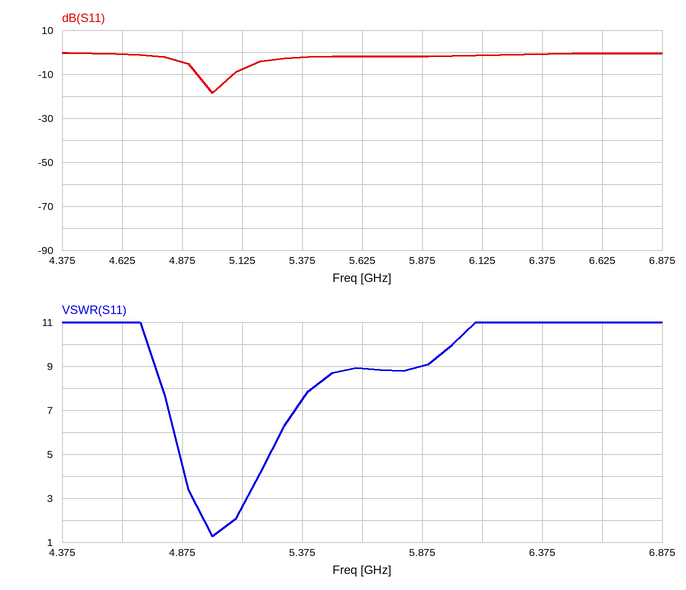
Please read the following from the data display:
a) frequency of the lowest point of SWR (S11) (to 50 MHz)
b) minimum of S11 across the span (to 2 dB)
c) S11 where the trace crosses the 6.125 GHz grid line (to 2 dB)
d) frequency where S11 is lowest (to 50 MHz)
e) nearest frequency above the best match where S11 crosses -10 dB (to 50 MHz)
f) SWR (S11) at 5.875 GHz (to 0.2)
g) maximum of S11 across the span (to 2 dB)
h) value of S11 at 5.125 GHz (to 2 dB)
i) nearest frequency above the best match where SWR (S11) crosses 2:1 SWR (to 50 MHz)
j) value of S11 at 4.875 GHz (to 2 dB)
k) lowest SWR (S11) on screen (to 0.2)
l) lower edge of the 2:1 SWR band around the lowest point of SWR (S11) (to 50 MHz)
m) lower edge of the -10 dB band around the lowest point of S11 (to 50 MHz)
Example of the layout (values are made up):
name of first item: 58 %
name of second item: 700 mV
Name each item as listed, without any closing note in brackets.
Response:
frequency of the lowest point of SWR (S11): 5.00 GHz
minimum of S11 across the span: -18 dB
S11 where the trace crosses the 6.125 GHz grid line: -2 dB
frequency where S11 is lowest: 5.00 GHz
nearest frequency above the best match where S11 crosses -10 dB: 5.10 GHz
SWR (S11) at 5.875 GHz: 9.0
maximum of S11 across the span: 0 dB
value of S11 at 5.125 GHz: -8 dB
nearest frequency above the best match where SWR (S11) crosses 2:1 SWR: 5.10 GHz
value of S11 at 4.875 GHz: -4 dB
lowest SWR (S11) on screen: 1.2
lower edge of the 2:1 SWR band around the lowest point of SWR (S11): 4.95 GHz
lower edge of the -10 dB band around the lowest point of S11: 4.95 GHz
